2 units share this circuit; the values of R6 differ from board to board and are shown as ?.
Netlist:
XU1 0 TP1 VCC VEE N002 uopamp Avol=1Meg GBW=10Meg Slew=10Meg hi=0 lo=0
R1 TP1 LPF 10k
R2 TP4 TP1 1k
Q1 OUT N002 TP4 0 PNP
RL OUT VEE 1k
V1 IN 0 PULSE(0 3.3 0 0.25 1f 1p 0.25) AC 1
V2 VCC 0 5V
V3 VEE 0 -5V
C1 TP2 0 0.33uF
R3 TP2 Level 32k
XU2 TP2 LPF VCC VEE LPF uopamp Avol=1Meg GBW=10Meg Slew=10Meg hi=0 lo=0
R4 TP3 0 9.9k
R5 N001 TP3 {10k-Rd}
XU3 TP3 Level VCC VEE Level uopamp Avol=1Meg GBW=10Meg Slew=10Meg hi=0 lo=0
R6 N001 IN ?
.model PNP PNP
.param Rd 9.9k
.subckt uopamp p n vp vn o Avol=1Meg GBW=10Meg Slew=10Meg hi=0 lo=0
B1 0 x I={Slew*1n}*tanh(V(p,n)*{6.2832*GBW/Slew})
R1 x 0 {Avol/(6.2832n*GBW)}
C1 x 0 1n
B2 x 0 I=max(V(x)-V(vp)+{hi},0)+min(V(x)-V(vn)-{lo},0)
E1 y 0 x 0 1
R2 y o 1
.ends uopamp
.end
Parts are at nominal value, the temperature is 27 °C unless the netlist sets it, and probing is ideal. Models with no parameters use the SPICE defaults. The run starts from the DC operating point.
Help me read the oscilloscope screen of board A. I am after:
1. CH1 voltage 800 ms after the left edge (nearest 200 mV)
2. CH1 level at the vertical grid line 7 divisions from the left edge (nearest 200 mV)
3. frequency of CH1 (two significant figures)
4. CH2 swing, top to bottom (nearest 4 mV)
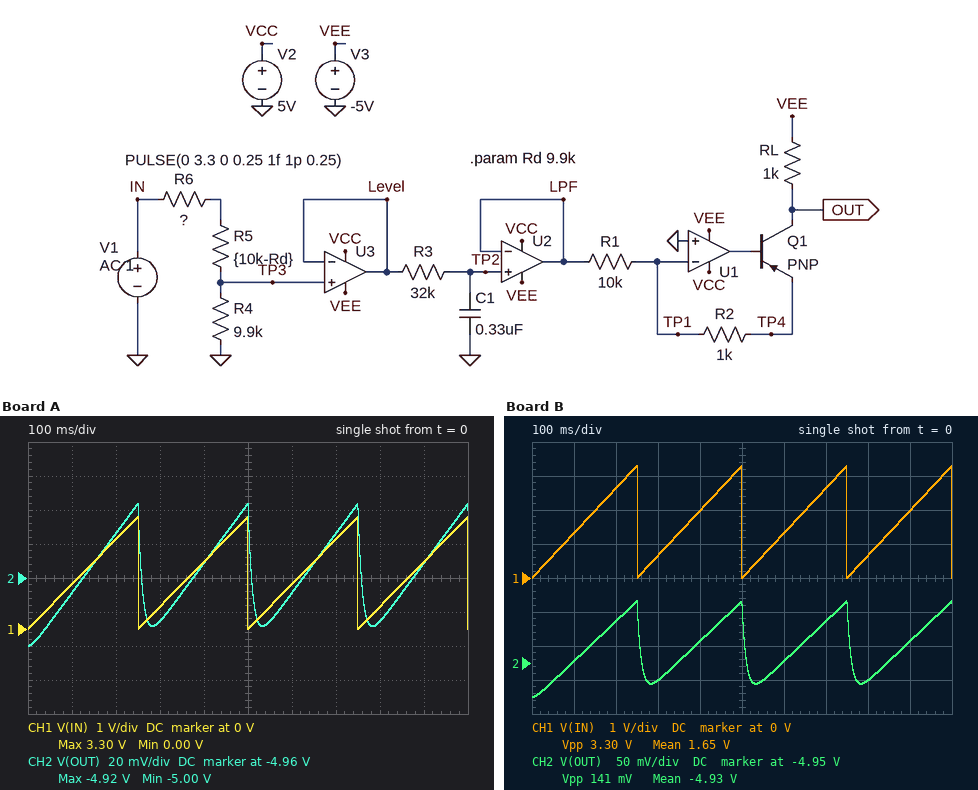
600 mV
2.6 V
4.0 Hz
84 mV
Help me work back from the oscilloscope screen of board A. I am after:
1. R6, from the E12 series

27 kΩ
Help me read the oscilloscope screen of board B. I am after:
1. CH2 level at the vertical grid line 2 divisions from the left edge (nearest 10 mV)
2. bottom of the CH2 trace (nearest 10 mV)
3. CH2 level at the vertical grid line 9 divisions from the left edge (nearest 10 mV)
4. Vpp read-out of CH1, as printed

-4.89 V
-5.00 V
-4.92 V
3.30 V
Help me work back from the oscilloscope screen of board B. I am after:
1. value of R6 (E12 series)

12 kΩ
